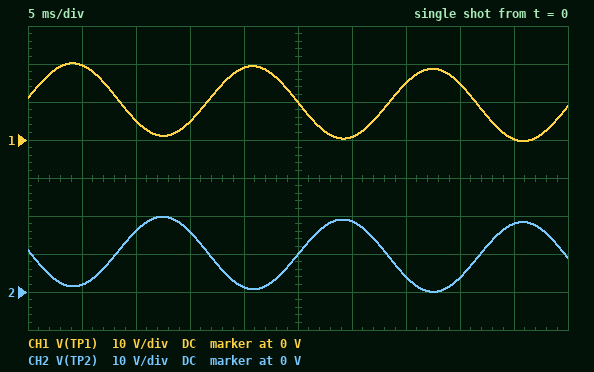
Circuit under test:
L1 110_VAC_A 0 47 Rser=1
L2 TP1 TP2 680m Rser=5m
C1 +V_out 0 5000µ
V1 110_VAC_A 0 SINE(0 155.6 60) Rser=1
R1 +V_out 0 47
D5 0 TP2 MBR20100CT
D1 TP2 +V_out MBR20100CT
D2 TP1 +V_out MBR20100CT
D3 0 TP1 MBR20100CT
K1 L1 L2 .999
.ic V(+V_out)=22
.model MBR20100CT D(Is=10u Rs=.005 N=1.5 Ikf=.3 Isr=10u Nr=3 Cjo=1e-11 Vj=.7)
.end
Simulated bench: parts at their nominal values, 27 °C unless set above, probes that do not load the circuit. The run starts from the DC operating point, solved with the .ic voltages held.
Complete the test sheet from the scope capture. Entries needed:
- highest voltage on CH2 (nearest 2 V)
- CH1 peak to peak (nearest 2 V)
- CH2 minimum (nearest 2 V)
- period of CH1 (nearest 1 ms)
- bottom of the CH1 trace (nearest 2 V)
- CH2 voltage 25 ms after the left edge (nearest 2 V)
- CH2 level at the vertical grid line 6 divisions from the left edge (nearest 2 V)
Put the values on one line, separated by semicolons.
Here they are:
20 V; 20 V; 0 V; 17 ms; 0 V; 10 V; 18 V
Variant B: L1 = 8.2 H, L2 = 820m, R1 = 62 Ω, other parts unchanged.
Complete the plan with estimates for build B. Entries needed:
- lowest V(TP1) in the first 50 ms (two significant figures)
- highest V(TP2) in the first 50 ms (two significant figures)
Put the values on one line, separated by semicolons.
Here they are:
-610 mV; 45 V
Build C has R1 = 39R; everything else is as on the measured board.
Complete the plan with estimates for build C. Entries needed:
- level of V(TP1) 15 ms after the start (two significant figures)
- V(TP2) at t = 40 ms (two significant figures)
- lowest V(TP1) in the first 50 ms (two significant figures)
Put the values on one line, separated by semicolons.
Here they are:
4.7 V; 3.5 V; -440 mV
